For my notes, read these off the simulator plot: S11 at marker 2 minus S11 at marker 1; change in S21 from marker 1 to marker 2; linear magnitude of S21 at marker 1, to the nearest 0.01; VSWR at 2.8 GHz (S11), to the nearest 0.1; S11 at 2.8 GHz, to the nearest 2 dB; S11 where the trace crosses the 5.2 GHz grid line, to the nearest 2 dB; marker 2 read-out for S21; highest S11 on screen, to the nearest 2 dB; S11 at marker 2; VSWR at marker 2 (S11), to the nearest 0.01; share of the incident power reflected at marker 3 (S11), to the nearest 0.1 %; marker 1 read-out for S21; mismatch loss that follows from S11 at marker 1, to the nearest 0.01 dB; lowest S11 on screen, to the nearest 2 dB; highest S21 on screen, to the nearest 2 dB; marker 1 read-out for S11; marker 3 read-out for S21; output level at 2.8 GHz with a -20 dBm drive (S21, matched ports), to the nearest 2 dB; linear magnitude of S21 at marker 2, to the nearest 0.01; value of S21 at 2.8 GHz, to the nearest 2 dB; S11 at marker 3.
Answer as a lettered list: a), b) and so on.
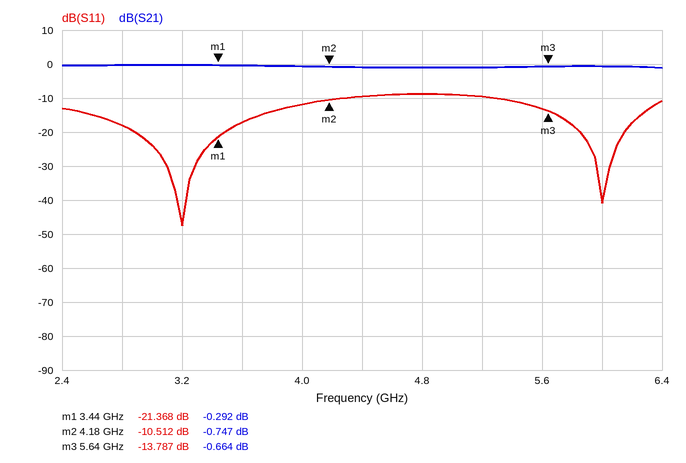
a) 10.856 dB
b) -0.455 dB
c) 0.97
d) 1.3
e) -18 dB
f) -10 dB
g) -0.747 dB
h) -8 dB
i) -10.512 dB
j) 1.85
k) 4.2 %
l) -0.292 dB
m) 0.03 dB
n) -48 dB
o) 0 dB
p) -21.368 dB
q) -0.664 dB
r) -20 dBm
s) 0.92
t) 0 dB
u) -13.787 dB
